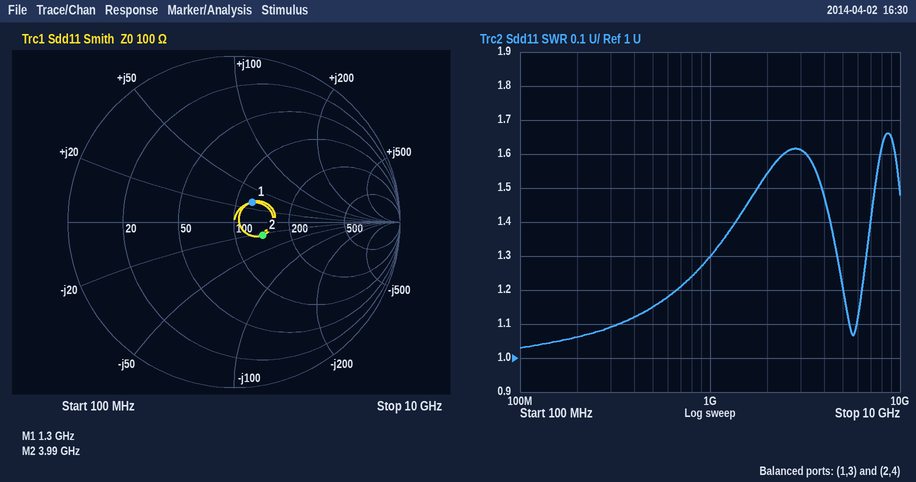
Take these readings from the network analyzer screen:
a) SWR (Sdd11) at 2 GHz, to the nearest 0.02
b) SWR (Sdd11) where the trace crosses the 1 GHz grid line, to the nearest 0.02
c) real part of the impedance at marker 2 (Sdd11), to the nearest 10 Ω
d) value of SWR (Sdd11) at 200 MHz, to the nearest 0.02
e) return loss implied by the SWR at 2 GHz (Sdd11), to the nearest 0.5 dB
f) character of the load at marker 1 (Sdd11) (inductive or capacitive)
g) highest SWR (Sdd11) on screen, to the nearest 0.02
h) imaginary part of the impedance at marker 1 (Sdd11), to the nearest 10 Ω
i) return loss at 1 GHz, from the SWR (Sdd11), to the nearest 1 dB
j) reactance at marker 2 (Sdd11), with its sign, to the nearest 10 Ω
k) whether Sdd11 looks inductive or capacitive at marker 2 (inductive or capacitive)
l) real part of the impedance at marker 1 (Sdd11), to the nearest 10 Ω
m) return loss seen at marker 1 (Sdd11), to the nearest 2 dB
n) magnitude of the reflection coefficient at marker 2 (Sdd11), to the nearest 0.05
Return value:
1.54
1.30
140 Ω
1.06
13.5 dB
inductive
1.66
+30 Ω
18 dB
-20 Ω
capacitive
120 Ω
16 dB
0.20
